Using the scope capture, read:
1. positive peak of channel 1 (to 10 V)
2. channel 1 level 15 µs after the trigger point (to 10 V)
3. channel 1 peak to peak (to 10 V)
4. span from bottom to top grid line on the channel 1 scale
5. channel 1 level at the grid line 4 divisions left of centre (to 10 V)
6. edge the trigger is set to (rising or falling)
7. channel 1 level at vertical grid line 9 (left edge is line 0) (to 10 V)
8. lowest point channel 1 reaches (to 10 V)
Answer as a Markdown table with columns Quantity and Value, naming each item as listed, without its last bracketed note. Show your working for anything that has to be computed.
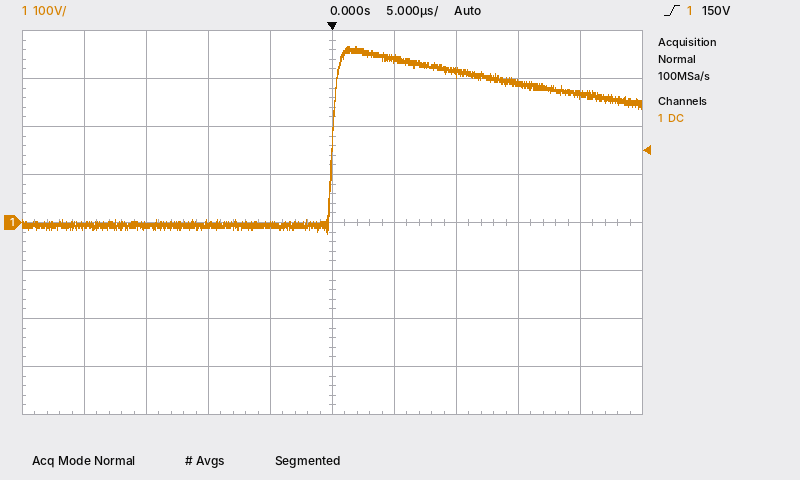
| Quantity | Value |
|---|---|
| positive peak of channel 1 | 370 V |
| channel 1 level 15 µs after the trigger point | 290 V |
| channel 1 peak to peak | 370 V − (-20 V) = 390 V |
| span from bottom to top grid line on the channel 1 scale | 800 V |
| channel 1 level at the grid line 4 divisions left of centre | -10 V |
| edge the trigger is set to | rising |
| channel 1 level at vertical grid line 9 (left edge is line 0) | 270 V |
| lowest point channel 1 reaches | -20 V |
